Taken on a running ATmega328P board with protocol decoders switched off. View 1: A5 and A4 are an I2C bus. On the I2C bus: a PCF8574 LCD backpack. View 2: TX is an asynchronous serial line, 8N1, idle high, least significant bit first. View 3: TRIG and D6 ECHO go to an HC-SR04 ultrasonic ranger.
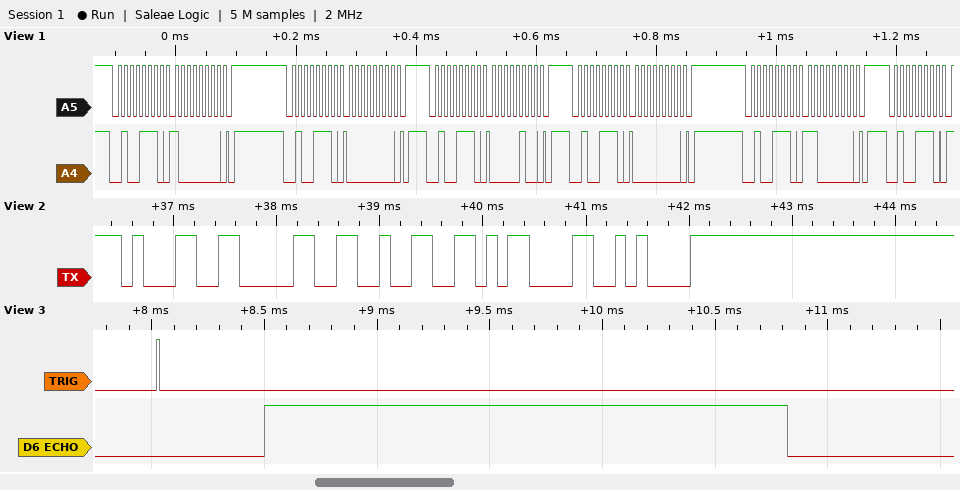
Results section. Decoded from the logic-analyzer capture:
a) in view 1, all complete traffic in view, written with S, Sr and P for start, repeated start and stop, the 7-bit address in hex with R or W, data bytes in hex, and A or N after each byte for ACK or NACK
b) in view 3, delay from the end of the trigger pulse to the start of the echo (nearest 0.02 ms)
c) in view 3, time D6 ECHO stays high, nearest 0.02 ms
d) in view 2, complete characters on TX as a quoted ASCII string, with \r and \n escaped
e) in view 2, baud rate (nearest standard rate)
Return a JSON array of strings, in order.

["S 27W A 80 A P S 27W A 00 A P S 27W A 04 A P S 27W A 00 A P S 27W A C0 A P S 27W A", "0.46 ms", "2.32 ms", "\"102\\r\\n\"", "9600 baud"]
